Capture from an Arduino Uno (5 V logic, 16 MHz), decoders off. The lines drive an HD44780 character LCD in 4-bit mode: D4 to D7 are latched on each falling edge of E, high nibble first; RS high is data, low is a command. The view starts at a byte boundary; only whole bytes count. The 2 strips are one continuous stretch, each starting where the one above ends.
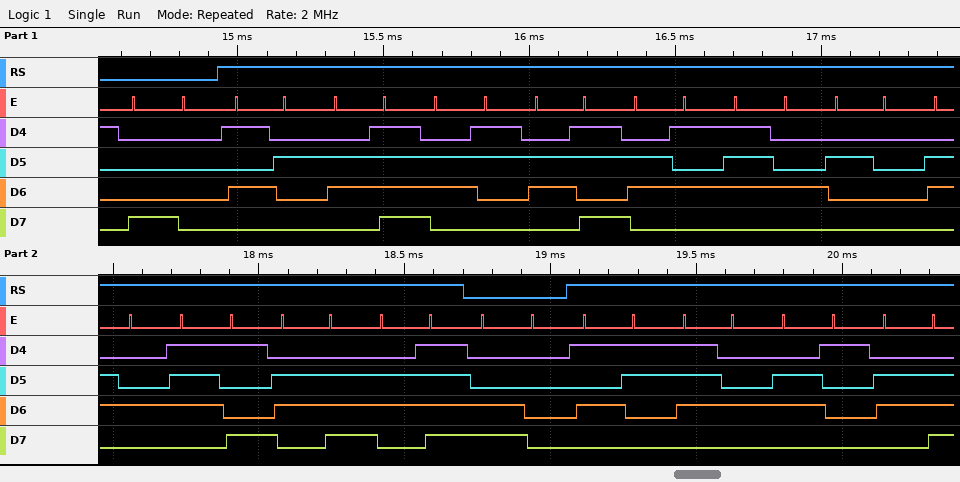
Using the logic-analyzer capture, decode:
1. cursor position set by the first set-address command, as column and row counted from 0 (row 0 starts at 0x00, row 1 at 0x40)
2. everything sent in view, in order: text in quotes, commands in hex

column 0, row 0
0x80 "Rocket dyno" 0xC0 "Stan"
